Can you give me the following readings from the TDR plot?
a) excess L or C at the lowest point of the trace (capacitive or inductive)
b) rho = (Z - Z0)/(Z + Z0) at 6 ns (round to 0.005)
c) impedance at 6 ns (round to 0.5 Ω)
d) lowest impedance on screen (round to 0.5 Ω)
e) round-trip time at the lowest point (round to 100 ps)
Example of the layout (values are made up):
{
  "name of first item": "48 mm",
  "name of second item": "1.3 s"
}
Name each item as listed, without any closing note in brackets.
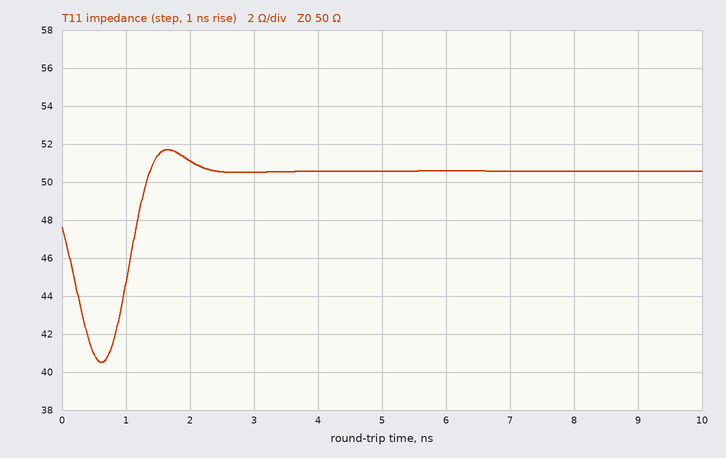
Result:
{
  "excess L or C at the lowest point of the trace": "capacitive",
  "rho = (Z - Z0)/(Z + Z0) at 6 ns": "+0.005",
  "impedance at 6 ns": "50.5 Ω",
  "lowest impedance on screen": "40.5 Ω",
  "round-trip time at the lowest point": "600 ps"
}
